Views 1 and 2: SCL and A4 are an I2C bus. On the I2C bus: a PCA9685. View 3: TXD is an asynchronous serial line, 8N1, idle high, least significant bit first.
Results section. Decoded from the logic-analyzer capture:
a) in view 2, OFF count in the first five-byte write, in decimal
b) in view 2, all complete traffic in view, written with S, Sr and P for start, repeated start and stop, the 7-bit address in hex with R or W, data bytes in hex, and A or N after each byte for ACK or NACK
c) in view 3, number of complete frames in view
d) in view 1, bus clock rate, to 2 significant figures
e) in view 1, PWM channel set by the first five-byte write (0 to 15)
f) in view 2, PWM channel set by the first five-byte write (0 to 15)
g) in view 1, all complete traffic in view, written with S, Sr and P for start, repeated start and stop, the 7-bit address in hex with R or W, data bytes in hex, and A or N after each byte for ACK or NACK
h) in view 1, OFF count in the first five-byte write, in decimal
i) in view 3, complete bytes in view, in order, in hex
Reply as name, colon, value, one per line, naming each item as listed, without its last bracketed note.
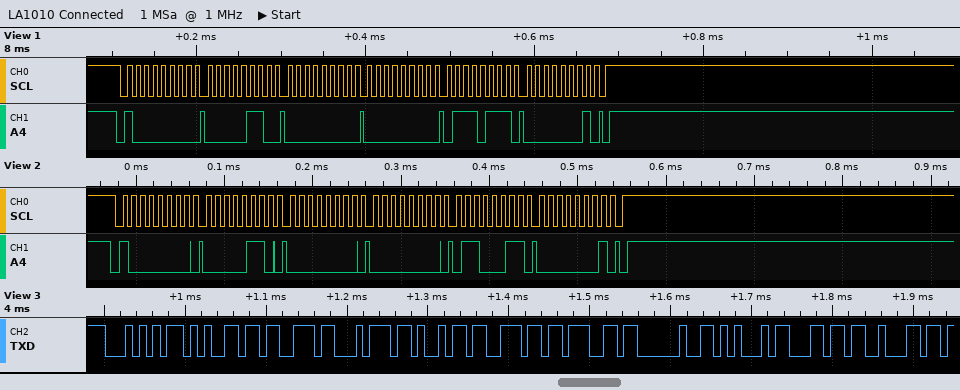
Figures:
in view 2, OFF count in the first five-byte write, in decimal: 355
in view 2, all complete traffic in view, written with S, Sr and P for start, repeated start and stop, the 7-bit address in hex with R or W, data bytes in hex, and A or N after each byte for ACK or NACK: S 40W A 06 A 00 A 00 A 63 A 01 A P
in view 3, number of complete frames in view: 11
in view 1, bus clock rate, to 2 significant figures: 100 kHz
in view 1, PWM channel set by the first five-byte write: 0
in view 2, PWM channel set by the first five-byte write: 0
in view 1, all complete traffic in view, written with S, Sr and P for start, repeated start and stop, the 7-bit address in hex with R or W, data bytes in hex, and A or N after each byte for ACK or NACK: S 40W A 06 A 00 A 00 A 77 A 01 A P
in view 1, OFF count in the first five-byte write, in decimal: 375
in view 3, complete bytes in view, in order, in hex: 54 65 73 74 69 6E 67 20 45 6C 62
